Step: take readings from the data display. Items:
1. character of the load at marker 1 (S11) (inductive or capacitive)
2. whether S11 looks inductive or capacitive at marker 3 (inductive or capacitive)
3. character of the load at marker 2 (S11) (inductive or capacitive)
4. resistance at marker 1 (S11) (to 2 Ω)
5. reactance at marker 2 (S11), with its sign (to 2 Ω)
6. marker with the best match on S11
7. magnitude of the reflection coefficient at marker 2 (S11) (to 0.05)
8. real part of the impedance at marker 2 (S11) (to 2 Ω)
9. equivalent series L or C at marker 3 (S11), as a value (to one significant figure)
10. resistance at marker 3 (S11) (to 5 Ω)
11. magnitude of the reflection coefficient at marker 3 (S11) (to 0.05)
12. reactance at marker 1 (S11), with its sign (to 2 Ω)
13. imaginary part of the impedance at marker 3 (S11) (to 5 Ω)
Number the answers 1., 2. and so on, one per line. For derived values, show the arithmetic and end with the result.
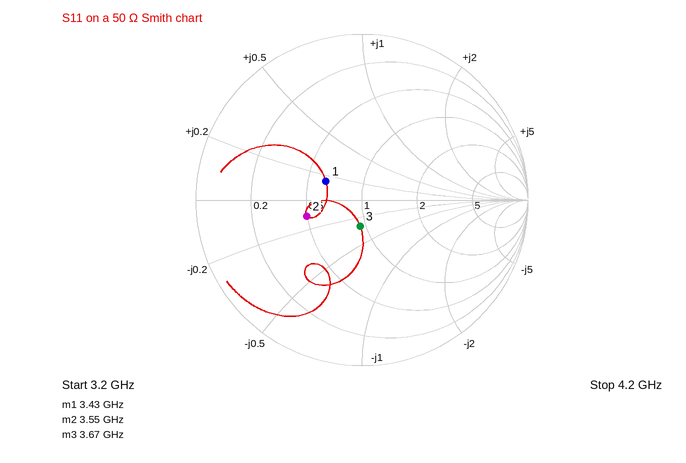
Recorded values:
1. inductive
2. capacitive
3. capacitive
4. 32 Ω
5. -6 Ω
6. marker 3
7. 0.35
8. 24 Ω
9. C = 1/(2π × 3.67 GHz × 15 Ω) ≈ 3 pF
10. 45 Ω
11. 0.15
12. +8 Ω
13. -15 Ω
